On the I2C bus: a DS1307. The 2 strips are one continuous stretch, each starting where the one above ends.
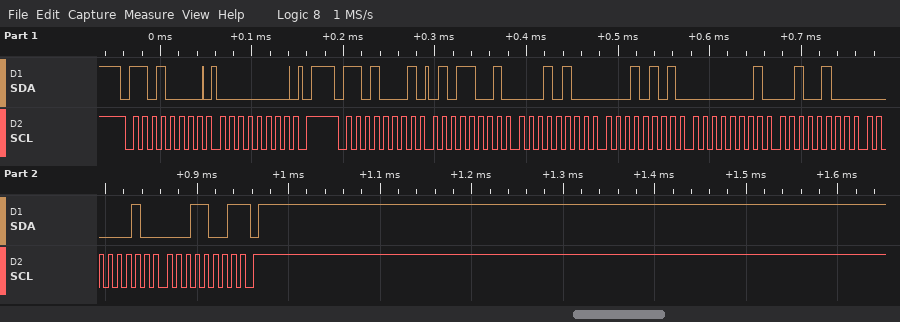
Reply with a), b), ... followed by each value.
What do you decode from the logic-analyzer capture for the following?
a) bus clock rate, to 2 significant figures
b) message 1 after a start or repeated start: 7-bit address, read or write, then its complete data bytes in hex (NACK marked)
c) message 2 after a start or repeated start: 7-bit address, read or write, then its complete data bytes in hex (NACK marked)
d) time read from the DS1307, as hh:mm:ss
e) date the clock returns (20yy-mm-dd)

a) 100 kHz
b) 0x68 write: 00
c) 0x68 read: 59 14 15 01 24 02 19 NACK
d) 15:14:59
e) 2019-02-24
